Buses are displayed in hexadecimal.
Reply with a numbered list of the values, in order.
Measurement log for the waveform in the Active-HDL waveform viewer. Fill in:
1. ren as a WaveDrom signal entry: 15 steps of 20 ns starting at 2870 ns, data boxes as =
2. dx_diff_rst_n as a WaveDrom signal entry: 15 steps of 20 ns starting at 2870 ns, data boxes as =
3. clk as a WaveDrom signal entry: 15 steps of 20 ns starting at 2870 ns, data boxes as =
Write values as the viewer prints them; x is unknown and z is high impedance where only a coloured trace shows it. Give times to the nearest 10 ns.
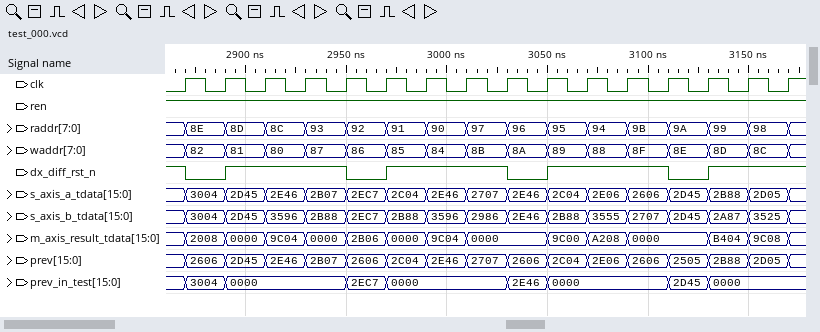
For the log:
1. {name: 'ren', wave: '1..............'}
2. {name: 'dx_diff_rst_n', wave: '01..01..01..01.'}
3. {name: 'clk', wave: 'p..............'}
